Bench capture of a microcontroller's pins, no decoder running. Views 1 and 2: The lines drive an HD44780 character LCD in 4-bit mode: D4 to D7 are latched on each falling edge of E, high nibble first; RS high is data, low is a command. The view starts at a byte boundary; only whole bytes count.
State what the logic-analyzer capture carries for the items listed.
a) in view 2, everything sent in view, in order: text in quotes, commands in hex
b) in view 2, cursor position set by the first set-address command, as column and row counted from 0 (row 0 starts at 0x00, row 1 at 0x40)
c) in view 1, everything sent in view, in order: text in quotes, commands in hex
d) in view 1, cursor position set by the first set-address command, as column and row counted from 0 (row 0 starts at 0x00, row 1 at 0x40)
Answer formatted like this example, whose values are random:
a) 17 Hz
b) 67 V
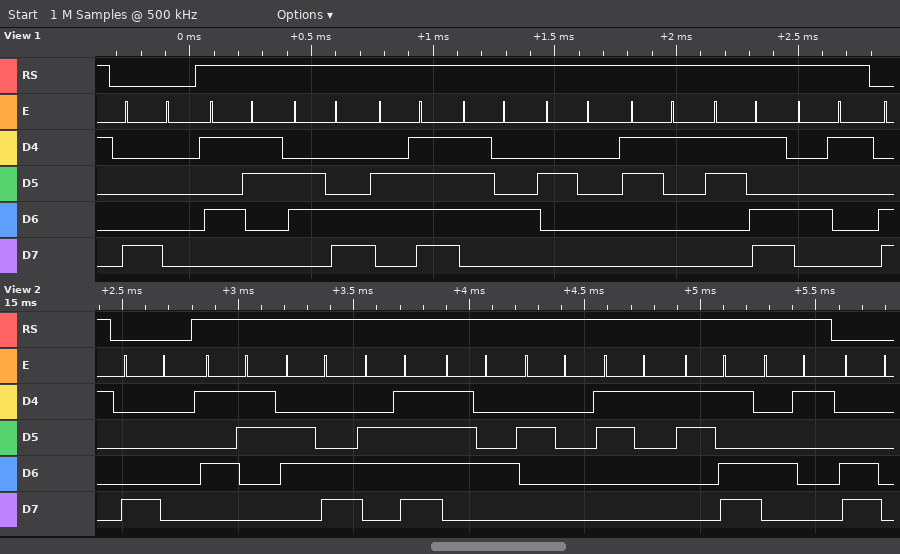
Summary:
a) 0x80 "Slot 1=A" 0xC0
b) column 0, row 0
c) 0x80 "Slot 1=A"
d) column 0, row 0
